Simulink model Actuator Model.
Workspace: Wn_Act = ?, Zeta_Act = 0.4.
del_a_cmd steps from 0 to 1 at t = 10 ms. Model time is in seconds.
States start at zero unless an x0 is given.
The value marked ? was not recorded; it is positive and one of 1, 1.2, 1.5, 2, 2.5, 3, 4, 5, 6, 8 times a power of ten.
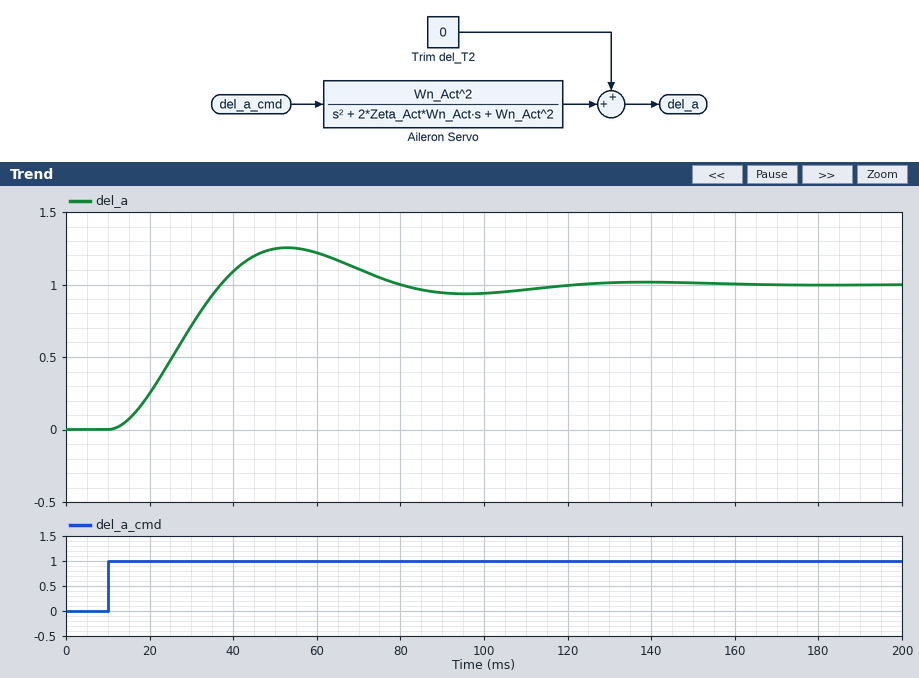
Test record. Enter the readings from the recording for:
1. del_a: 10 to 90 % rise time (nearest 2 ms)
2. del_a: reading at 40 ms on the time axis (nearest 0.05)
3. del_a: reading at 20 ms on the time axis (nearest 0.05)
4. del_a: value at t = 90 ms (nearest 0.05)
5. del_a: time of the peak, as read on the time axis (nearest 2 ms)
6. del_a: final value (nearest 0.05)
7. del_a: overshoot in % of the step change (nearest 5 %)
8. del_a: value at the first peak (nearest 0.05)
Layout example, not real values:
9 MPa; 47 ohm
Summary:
18 ms; 1.10; 0.25; 0.95; 52 ms; 1.00; 25 %; 1.25
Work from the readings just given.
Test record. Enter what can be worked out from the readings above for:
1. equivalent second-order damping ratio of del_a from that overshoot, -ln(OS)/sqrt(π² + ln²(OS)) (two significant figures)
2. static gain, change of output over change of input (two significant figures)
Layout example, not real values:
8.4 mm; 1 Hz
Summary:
0.40; 1.0
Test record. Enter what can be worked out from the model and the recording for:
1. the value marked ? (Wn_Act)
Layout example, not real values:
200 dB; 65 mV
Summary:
80
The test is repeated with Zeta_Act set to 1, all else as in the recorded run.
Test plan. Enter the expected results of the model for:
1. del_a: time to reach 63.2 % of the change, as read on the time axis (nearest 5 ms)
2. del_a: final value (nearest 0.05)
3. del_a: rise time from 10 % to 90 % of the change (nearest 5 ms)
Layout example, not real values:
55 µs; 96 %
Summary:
35 ms; 1.00; 40 ms
